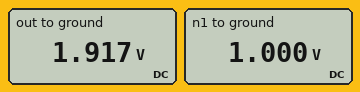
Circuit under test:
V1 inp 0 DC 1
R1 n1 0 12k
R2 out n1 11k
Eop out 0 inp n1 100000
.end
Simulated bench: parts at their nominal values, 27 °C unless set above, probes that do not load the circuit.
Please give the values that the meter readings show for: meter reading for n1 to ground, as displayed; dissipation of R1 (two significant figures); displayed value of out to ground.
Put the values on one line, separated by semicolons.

1.000 V; 83 µW; 1.917 V
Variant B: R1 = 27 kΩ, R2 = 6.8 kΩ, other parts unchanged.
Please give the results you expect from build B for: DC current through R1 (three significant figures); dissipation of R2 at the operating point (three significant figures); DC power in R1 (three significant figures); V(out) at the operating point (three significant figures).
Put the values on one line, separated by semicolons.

37.0 µA; 9.33 µW; 37.0 µW; 1.25 V
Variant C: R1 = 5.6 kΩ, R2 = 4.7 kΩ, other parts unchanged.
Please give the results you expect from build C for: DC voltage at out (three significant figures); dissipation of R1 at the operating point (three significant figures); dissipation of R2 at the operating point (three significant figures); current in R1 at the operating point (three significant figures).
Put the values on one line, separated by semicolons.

1.84 V; 179 µW; 150 µW; 179 µA
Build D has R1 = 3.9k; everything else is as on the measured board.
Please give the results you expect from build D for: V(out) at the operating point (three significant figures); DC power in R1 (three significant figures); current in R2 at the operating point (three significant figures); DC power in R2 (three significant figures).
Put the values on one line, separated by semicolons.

3.82 V; 256 µW; 256 µA; 723 µW
